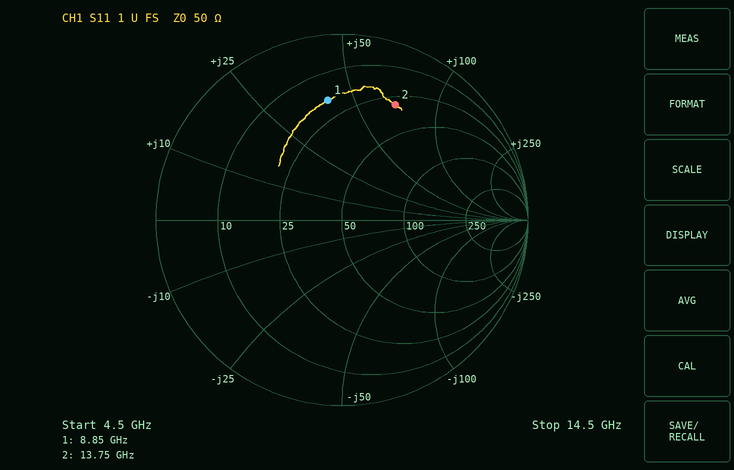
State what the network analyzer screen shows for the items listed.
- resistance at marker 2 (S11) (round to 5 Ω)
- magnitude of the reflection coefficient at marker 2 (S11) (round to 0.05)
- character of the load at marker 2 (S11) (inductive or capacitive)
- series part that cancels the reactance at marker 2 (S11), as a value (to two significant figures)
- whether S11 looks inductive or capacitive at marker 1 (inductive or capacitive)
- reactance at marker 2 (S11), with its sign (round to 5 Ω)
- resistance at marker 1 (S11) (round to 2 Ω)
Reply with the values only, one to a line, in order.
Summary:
30 Ω
0.70
inductive
170 fF
inductive
+70 Ω
18 Ω
